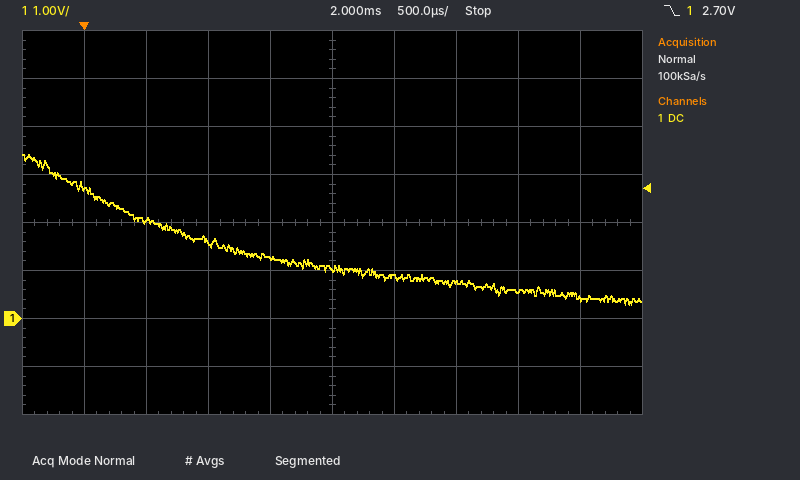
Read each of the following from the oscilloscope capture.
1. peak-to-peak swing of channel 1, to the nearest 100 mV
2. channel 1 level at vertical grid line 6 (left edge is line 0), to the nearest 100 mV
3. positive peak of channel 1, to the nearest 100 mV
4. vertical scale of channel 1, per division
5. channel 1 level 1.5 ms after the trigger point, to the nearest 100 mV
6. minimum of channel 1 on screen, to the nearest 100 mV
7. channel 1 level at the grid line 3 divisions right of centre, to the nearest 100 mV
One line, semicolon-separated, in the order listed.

3.1 V; 900 mV; 3.4 V; 1 V; 1.3 V; 300 mV; 600 mV
